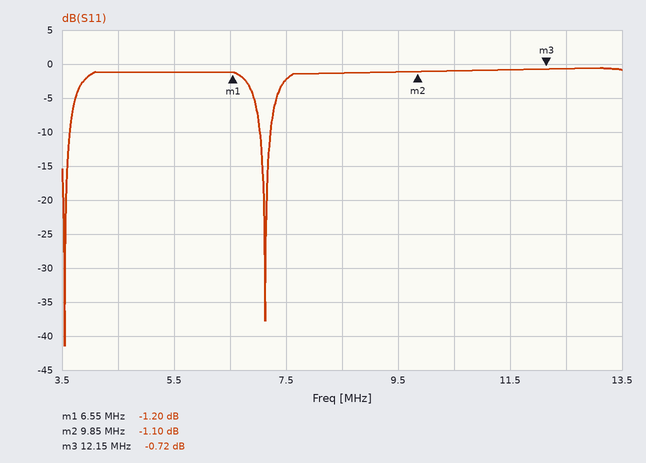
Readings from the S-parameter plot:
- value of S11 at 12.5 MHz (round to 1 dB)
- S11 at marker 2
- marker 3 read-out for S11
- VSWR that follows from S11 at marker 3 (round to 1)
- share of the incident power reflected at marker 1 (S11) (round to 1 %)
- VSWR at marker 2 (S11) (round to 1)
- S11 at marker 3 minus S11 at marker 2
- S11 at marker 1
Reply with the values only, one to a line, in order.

-1 dB
-1.10 dB
-0.72 dB
24
76 %
16
0.38 dB
-1.20 dB
